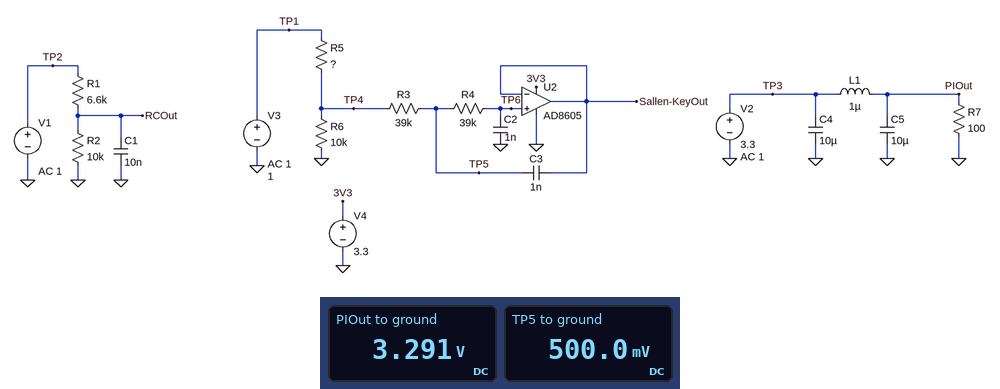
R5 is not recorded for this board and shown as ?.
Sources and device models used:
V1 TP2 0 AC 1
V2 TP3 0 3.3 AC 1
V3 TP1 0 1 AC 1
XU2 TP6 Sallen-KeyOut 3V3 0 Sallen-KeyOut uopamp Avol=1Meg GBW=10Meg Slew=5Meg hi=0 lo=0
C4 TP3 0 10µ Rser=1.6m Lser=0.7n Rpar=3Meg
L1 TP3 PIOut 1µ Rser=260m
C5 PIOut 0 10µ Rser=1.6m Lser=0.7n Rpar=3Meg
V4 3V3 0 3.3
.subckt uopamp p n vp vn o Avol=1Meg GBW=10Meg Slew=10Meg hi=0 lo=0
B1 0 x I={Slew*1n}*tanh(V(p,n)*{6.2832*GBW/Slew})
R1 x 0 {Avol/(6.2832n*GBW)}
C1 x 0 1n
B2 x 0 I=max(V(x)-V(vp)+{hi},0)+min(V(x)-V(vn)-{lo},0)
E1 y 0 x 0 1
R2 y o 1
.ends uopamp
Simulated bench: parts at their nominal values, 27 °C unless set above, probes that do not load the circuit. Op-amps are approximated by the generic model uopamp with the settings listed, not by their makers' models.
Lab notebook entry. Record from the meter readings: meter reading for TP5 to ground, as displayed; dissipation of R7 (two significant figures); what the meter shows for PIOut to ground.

500.0 mV
110 mW
3.291 V
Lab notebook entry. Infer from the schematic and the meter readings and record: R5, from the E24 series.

10 kΩ
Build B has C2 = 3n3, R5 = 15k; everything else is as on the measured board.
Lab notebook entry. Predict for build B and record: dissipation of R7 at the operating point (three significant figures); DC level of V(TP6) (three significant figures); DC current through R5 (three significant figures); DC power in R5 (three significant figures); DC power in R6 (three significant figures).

108 mW
400 mV
40.0 µA
24.0 µW
16.0 µW
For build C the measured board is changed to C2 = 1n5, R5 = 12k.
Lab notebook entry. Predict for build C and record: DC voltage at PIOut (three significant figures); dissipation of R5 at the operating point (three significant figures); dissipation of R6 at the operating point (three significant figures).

3.29 V
24.8 µW
20.7 µW
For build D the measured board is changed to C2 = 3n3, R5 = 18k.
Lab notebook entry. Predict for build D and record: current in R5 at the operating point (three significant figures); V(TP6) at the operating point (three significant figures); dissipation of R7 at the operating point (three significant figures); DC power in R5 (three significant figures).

35.7 µA
357 mV
108 mW
23.0 µW
